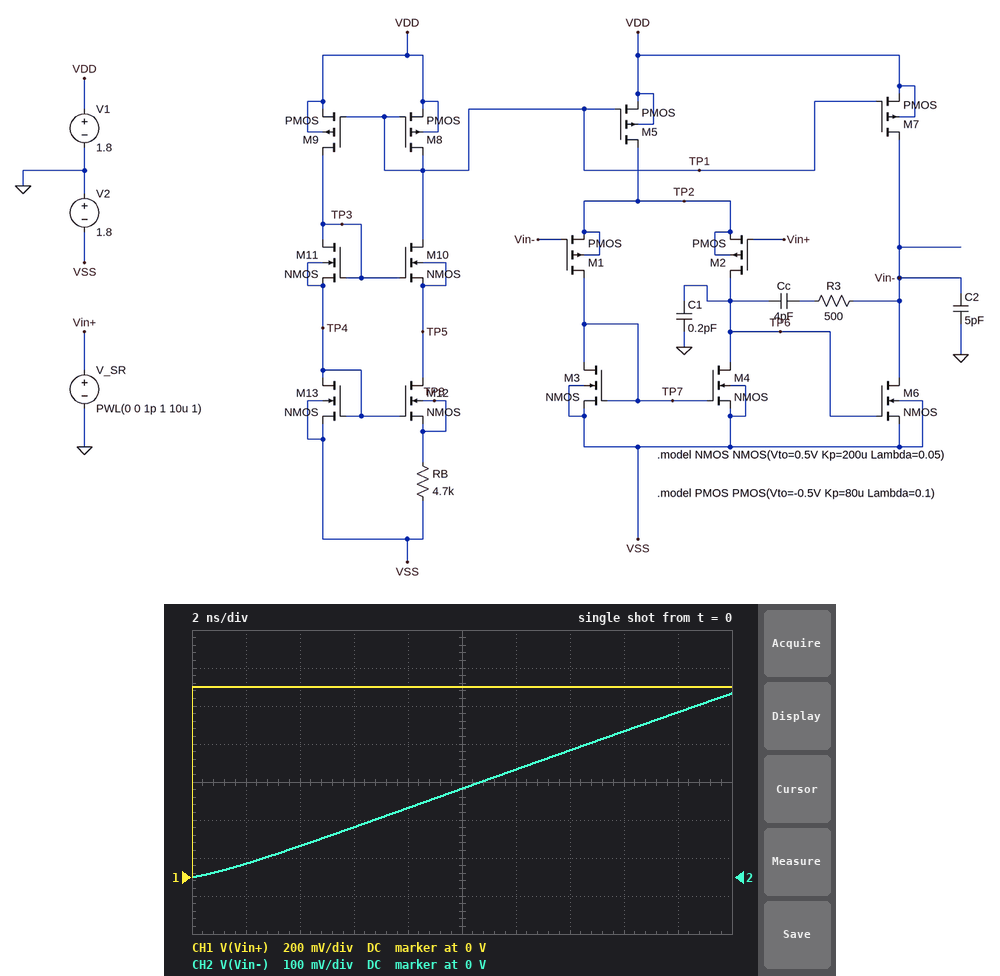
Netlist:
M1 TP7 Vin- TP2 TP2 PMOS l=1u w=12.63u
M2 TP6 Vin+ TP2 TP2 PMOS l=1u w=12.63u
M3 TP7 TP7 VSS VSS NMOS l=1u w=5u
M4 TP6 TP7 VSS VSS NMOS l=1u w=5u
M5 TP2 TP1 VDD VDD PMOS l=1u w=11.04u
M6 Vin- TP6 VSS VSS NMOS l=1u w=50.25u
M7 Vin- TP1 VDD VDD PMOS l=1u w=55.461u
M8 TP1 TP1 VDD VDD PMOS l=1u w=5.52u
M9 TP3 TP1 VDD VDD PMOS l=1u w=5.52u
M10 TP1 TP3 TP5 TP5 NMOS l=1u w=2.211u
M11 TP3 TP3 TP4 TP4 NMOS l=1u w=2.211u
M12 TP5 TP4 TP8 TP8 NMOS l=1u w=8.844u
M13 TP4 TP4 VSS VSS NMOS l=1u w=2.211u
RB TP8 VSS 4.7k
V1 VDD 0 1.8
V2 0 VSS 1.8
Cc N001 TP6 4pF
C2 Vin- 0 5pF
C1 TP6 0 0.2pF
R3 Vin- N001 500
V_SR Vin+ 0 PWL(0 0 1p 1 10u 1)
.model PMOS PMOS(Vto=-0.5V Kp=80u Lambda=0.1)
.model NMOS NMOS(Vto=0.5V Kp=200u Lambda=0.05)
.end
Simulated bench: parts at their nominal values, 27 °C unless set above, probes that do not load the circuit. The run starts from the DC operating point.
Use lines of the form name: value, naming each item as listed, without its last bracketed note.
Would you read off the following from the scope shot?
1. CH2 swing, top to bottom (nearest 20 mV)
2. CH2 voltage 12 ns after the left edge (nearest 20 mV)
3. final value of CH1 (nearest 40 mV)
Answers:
CH2 swing, top to bottom: 480 mV
CH2 voltage 12 ns after the left edge: 280 mV
final value of CH1: 1.00 V
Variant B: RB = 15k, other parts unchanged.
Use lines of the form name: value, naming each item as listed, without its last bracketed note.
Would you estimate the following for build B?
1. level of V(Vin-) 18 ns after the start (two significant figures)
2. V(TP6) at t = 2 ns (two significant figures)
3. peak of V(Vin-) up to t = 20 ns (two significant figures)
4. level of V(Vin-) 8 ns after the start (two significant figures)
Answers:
level of V(Vin-) 18 ns after the start: 38 mV
V(TP6) at t = 2 ns: -1.2 V
peak of V(Vin-) up to t = 20 ns: 44 mV
level of V(Vin-) 8 ns after the start: 9.4 mV
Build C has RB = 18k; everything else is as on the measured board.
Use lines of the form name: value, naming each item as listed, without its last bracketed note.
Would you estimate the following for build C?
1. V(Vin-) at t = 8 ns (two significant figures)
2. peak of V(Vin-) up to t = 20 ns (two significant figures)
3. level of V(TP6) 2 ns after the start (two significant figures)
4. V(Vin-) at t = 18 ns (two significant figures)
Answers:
V(Vin-) at t = 8 ns: 4.8 mV
peak of V(Vin-) up to t = 20 ns: 28 mV
level of V(TP6) 2 ns after the start: -1.2 V
V(Vin-) at t = 18 ns: 24 mV
